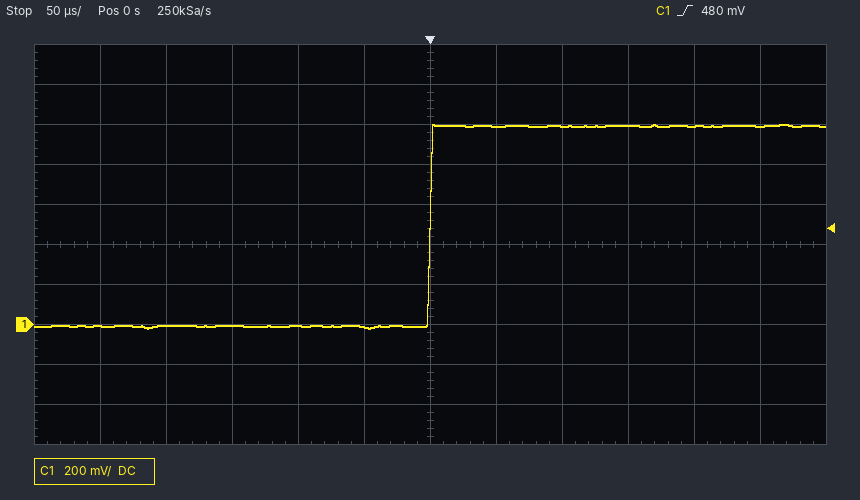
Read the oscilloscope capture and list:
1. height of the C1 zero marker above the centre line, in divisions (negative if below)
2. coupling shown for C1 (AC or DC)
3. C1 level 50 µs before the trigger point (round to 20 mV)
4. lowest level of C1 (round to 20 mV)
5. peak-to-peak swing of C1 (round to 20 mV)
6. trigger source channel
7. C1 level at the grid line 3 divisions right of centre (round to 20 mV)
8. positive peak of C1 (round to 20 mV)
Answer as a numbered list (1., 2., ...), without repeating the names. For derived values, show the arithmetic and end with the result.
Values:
1. -2.0 div
2. DC
3. -20 mV
4. -20 mV
5. 1.00 V − (-20 mV) = 1.02 V
6. C1
7. 1.00 V
8. 1.00 V
